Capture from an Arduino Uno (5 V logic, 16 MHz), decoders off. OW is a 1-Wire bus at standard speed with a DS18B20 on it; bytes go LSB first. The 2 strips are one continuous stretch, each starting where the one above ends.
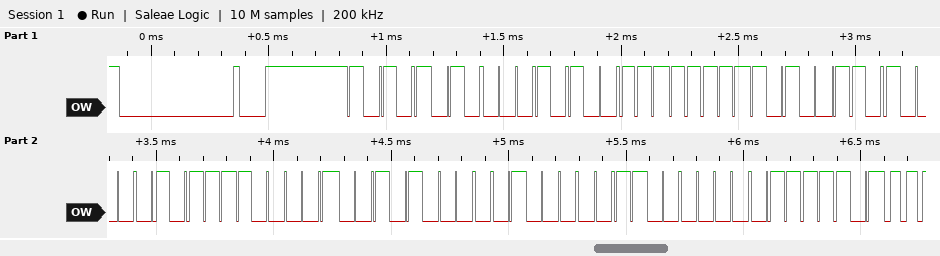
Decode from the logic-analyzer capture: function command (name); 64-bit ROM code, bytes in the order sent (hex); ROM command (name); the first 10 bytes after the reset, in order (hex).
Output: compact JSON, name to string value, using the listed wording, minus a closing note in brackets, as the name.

{"function command": "Read Scratchpad", "64-bit ROM code, bytes in the order sent": "28 FF 65 A1 87 14 04 03", "ROM command": "Match ROM", "the first 10 bytes after the reset, in order": "55 28 FF 65 A1 87 14 04 03 BE"}
